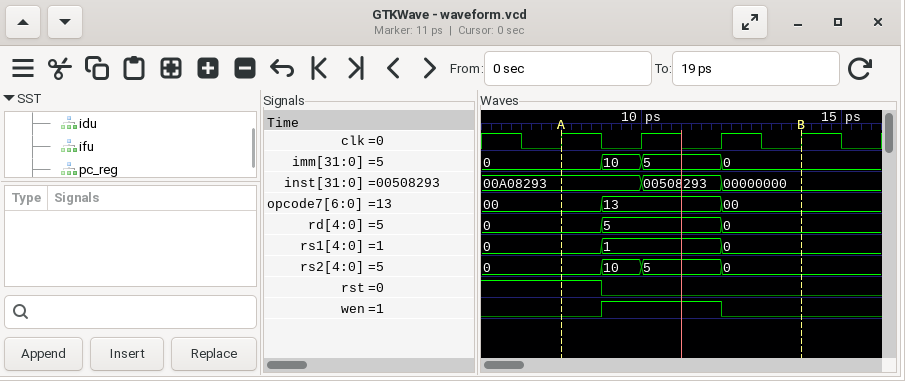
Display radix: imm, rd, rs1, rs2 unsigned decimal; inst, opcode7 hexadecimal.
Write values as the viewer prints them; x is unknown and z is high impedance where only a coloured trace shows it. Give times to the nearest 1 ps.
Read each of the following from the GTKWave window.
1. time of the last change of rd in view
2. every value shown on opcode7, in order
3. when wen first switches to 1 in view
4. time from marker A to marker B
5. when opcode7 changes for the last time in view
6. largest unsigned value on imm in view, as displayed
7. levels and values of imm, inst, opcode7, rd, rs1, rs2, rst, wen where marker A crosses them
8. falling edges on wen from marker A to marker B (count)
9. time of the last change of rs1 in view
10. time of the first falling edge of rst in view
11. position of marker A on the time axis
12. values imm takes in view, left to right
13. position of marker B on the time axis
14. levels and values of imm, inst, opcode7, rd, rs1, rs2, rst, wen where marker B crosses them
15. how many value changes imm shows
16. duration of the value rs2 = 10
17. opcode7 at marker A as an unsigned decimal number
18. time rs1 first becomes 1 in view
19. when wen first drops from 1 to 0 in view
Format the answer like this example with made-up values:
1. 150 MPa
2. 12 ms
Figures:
1. 12 ps
2. 00, 13, 00
3. 9 ps
4. 6 ps
5. 12 ps
6. 10
7. imm=0, inst=00A08293, opcode7=00, rd=0, rs1=0, rs2=0, rst=1, wen=0
8. 1
9. 12 ps
10. 9 ps
11. 8 ps
12. 0, 10, 5, 0
13. 14 ps
14. imm=0, inst=00000000, opcode7=00, rd=0, rs1=0, rs2=0, rst=0, wen=0
15. 3
16. 1 ps
17. 0
18. 9 ps
19. 12 ps
